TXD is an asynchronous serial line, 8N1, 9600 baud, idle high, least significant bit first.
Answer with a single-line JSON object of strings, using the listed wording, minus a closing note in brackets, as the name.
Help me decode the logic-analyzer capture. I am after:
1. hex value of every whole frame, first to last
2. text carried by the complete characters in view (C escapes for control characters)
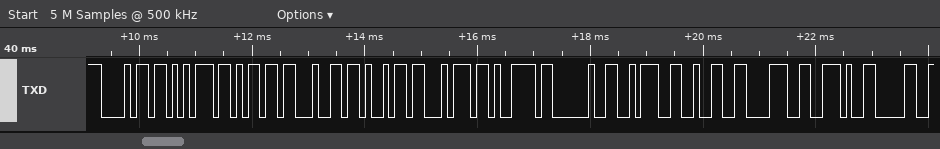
{"hex value of every whole frame, first to last": "68 75 6D 64 69 74 79 20 3A 32 38 2E 30", "text carried by the complete characters in view": "\"humdity :28.0\""}
